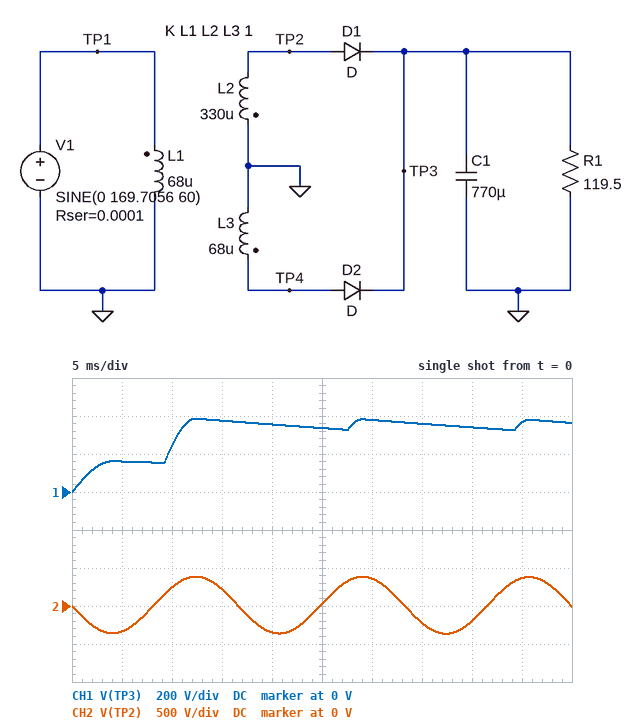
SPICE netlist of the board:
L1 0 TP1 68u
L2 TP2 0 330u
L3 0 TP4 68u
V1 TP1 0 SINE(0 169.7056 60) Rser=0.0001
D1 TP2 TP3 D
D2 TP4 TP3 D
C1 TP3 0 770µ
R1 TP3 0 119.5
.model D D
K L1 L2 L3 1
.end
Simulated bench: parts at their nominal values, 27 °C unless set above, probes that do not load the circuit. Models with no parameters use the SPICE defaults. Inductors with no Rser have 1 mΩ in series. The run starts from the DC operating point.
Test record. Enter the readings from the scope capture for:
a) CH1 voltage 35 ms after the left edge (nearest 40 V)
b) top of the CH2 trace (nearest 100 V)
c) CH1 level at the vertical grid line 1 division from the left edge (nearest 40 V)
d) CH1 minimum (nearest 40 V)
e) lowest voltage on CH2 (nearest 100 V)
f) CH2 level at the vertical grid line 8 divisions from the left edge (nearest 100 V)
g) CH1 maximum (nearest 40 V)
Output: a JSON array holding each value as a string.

["360 V", "400 V", "160 V", "0 V", "-400 V", "-200 V", "400 V"]
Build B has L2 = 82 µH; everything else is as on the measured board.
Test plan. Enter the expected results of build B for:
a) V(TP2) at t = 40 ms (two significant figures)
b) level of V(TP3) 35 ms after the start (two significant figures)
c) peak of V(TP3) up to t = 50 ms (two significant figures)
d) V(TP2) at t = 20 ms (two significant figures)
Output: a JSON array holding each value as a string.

["-99 V", "180 V", "190 V", "-170 V"]
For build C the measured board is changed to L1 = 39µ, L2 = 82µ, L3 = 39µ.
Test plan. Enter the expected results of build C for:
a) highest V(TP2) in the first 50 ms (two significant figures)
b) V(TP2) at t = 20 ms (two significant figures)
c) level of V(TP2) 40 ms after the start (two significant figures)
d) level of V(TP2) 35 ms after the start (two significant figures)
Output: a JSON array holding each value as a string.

["260 V", "-230 V", "-120 V", "-150 V"]
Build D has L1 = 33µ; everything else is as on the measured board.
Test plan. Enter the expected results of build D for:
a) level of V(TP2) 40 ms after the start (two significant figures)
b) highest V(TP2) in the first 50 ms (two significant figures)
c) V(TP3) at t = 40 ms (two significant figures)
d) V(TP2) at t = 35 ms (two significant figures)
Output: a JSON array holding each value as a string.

["-260 V", "570 V", "490 V", "-340 V"]
